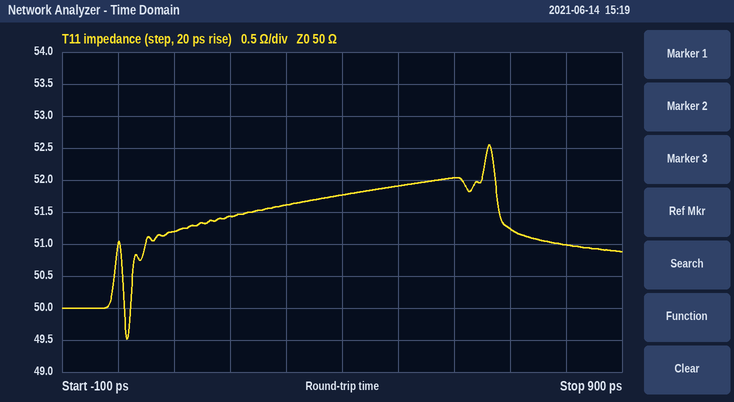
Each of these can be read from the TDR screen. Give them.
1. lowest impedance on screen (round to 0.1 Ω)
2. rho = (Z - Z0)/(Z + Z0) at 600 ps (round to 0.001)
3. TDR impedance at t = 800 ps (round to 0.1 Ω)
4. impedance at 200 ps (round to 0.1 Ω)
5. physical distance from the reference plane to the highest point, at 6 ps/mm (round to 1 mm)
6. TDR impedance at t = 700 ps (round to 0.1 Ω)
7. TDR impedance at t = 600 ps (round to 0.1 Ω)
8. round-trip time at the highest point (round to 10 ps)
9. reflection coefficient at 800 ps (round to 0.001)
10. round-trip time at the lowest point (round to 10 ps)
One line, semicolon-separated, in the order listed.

49.5 Ω; +0.020; 51.0 Ω; 51.4 Ω; 55 mm; 51.2 Ω; 52.0 Ω; 660 ps; +0.010; 20 ps
